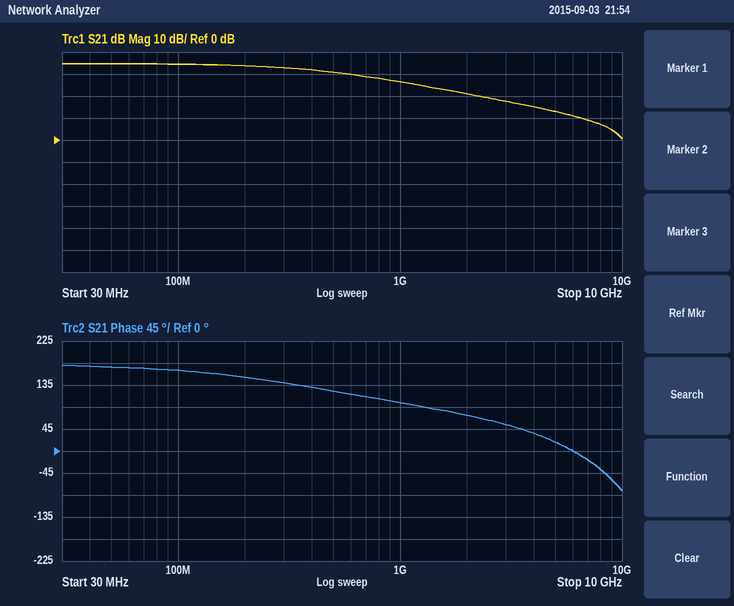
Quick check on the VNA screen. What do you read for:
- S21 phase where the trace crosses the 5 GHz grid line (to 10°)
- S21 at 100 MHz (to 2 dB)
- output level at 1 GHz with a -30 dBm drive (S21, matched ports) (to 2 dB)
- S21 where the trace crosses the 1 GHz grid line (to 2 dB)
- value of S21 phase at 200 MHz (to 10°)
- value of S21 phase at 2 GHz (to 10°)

20°
34 dB
-4 dBm
26 dB
150°
70°
